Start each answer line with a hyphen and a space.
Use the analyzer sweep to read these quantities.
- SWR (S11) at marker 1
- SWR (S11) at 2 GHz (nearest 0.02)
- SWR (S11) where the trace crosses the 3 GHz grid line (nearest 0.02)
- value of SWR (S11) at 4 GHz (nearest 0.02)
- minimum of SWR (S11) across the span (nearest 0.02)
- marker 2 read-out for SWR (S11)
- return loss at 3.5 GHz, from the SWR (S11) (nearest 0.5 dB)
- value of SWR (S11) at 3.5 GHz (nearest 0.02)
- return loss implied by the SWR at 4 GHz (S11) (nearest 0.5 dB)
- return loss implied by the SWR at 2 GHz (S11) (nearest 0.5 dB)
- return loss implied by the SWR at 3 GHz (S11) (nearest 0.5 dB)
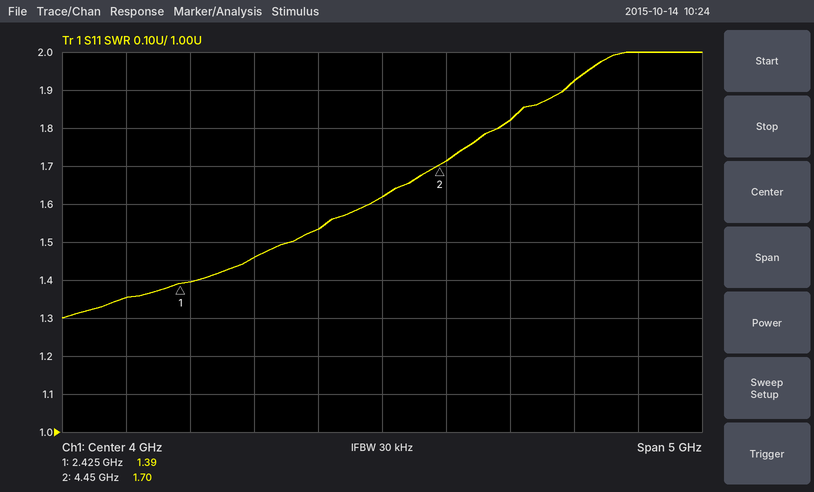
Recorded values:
- 1.39
- 1.36
- 1.46
- 1.62
- 1.30
- 1.70
- 13.5 dB
- 1.54
- 12.5 dB
- 16.5 dB
- 14.5 dB
